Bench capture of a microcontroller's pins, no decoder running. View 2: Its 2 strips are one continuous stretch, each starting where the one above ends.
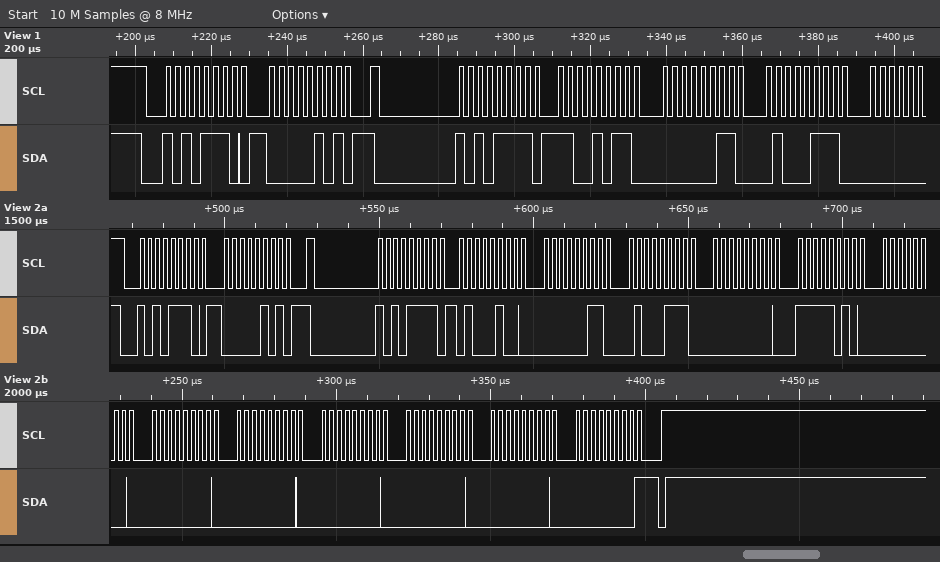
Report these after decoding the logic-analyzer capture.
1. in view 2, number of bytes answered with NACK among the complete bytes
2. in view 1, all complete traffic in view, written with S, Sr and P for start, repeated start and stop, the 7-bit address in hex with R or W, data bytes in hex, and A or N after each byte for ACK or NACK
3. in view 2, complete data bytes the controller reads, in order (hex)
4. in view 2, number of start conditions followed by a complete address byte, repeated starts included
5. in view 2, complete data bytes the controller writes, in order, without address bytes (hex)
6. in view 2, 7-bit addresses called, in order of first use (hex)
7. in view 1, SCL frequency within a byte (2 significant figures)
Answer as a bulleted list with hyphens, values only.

- 1
- S 57W A 05 A Sr 57R A CB A 03 A 47 A
- 44 03 47 00 FA 00 00 00 00 00 00 00
- 2
- 05
- 0x57
- 400 kHz
